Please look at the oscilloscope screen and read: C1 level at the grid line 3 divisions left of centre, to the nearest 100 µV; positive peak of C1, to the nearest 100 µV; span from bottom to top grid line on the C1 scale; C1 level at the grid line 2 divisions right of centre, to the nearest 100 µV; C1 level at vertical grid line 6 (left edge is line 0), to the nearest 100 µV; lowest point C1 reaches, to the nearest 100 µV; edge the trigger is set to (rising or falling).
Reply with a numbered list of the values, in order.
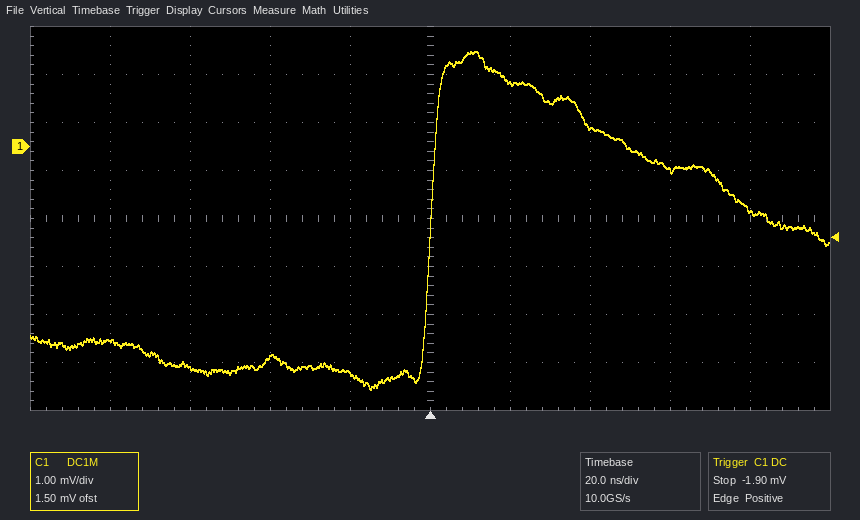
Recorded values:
1. -4.6 mV
2. 2.0 mV
3. 8 mV
4. 400 µV
5. 1.3 mV
6. -5.1 mV
7. rising
